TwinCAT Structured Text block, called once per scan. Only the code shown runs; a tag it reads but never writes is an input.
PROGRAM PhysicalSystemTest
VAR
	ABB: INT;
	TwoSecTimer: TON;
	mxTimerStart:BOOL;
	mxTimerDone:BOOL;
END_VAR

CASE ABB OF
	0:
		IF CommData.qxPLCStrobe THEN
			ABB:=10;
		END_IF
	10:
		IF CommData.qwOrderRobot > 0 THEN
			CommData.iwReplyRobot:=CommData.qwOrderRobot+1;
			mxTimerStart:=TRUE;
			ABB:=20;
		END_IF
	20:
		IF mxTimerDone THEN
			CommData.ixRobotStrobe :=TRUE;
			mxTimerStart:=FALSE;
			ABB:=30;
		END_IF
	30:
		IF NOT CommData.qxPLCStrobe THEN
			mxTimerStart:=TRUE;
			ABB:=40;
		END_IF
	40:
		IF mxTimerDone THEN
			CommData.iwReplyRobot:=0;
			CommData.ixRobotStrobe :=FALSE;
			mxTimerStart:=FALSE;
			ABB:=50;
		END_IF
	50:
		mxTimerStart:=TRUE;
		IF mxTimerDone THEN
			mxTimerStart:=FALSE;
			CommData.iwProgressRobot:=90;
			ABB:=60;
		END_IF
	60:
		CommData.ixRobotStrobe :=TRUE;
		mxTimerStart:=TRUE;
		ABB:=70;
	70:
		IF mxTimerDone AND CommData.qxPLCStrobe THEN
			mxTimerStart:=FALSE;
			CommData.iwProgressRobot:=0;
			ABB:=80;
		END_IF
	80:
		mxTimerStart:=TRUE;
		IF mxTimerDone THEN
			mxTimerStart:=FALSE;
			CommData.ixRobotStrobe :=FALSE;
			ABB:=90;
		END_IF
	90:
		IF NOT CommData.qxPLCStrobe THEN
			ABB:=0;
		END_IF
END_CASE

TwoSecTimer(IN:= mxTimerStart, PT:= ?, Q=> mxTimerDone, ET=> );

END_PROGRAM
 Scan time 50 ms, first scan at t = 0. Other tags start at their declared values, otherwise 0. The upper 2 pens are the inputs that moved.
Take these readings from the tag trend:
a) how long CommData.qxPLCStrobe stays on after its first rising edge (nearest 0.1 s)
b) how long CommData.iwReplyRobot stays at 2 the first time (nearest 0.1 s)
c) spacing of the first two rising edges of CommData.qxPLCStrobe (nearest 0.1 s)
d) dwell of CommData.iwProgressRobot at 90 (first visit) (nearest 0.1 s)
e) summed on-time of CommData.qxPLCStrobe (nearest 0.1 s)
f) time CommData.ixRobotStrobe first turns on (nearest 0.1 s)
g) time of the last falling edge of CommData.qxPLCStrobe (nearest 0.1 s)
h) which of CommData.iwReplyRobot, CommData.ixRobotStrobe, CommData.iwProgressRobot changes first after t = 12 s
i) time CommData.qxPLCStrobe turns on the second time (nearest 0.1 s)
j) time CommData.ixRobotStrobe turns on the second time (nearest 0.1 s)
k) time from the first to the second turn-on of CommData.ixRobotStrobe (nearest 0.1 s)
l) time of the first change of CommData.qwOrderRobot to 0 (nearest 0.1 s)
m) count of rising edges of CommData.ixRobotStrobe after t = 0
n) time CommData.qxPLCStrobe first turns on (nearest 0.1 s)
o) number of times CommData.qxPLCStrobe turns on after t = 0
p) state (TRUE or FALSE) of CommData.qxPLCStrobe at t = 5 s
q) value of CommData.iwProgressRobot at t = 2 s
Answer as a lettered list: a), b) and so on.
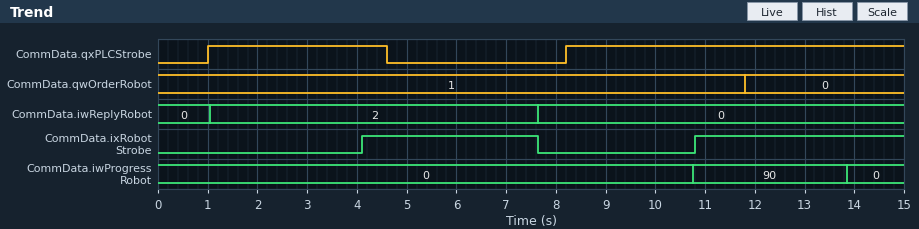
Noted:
a) 3.6 s
b) 6.6 s
c) 7.2 s
d) 3.1 s
e) 10.4 s
f) 4.1 s
g) 4.6 s
h) CommData.iwProgressRobot
i) 8.2 s
j) 10.8 s
k) 6.7 s
l) 11.8 s
m) 2
n) 1.0 s
o) 2
p) FALSE
q) 0
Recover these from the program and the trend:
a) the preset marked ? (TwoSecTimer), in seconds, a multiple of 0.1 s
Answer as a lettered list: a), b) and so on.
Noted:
a) 3.0 s
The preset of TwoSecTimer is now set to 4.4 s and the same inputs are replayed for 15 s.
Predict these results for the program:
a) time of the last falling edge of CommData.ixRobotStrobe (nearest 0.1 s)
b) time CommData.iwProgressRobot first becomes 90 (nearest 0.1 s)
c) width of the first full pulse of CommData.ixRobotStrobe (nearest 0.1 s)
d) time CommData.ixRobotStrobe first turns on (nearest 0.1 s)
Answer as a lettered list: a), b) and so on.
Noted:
a) 10.0 s
b) 14.5 s
c) 4.5 s
d) 5.5 s
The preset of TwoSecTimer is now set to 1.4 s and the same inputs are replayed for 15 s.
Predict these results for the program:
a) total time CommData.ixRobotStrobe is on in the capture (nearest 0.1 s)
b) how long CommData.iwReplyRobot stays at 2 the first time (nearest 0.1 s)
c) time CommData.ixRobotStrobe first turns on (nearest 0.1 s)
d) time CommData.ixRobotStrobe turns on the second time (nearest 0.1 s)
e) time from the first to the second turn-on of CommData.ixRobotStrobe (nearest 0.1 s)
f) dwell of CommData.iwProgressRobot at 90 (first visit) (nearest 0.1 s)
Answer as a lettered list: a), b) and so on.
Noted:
a) 6.5 s
b) 5.0 s
c) 2.5 s
d) 7.6 s
e) 5.1 s
f) 1.5 s
